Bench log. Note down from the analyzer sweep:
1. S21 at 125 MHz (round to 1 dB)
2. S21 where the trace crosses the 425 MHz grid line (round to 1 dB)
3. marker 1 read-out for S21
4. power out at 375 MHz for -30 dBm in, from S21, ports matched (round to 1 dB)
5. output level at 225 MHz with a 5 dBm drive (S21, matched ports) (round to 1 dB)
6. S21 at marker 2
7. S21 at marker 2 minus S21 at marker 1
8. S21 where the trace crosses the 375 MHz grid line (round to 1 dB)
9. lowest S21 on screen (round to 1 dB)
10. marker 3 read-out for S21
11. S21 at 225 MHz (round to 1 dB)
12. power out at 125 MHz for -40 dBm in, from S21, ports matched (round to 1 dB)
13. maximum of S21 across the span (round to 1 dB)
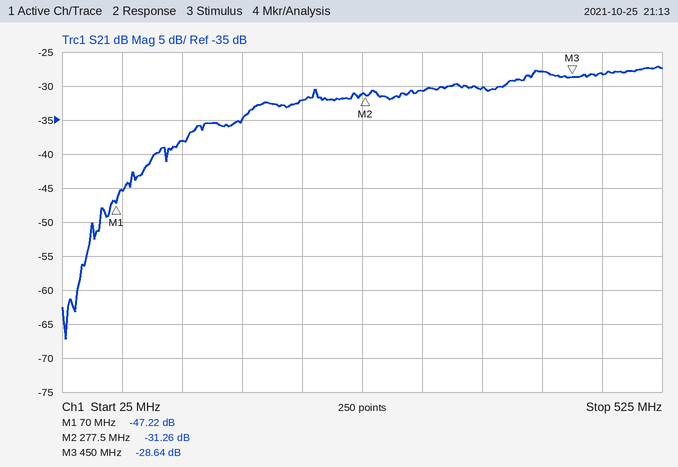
-38 dB
-28 dB
-47.22 dB
-60 dBm
-27 dBm
-31.26 dB
15.96 dB
-30 dB
-67 dB
-28.64 dB
-32 dB
-78 dBm
-27 dB
